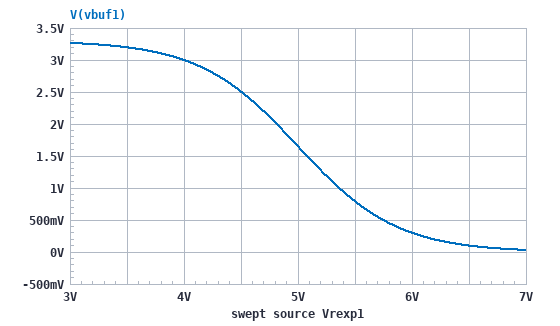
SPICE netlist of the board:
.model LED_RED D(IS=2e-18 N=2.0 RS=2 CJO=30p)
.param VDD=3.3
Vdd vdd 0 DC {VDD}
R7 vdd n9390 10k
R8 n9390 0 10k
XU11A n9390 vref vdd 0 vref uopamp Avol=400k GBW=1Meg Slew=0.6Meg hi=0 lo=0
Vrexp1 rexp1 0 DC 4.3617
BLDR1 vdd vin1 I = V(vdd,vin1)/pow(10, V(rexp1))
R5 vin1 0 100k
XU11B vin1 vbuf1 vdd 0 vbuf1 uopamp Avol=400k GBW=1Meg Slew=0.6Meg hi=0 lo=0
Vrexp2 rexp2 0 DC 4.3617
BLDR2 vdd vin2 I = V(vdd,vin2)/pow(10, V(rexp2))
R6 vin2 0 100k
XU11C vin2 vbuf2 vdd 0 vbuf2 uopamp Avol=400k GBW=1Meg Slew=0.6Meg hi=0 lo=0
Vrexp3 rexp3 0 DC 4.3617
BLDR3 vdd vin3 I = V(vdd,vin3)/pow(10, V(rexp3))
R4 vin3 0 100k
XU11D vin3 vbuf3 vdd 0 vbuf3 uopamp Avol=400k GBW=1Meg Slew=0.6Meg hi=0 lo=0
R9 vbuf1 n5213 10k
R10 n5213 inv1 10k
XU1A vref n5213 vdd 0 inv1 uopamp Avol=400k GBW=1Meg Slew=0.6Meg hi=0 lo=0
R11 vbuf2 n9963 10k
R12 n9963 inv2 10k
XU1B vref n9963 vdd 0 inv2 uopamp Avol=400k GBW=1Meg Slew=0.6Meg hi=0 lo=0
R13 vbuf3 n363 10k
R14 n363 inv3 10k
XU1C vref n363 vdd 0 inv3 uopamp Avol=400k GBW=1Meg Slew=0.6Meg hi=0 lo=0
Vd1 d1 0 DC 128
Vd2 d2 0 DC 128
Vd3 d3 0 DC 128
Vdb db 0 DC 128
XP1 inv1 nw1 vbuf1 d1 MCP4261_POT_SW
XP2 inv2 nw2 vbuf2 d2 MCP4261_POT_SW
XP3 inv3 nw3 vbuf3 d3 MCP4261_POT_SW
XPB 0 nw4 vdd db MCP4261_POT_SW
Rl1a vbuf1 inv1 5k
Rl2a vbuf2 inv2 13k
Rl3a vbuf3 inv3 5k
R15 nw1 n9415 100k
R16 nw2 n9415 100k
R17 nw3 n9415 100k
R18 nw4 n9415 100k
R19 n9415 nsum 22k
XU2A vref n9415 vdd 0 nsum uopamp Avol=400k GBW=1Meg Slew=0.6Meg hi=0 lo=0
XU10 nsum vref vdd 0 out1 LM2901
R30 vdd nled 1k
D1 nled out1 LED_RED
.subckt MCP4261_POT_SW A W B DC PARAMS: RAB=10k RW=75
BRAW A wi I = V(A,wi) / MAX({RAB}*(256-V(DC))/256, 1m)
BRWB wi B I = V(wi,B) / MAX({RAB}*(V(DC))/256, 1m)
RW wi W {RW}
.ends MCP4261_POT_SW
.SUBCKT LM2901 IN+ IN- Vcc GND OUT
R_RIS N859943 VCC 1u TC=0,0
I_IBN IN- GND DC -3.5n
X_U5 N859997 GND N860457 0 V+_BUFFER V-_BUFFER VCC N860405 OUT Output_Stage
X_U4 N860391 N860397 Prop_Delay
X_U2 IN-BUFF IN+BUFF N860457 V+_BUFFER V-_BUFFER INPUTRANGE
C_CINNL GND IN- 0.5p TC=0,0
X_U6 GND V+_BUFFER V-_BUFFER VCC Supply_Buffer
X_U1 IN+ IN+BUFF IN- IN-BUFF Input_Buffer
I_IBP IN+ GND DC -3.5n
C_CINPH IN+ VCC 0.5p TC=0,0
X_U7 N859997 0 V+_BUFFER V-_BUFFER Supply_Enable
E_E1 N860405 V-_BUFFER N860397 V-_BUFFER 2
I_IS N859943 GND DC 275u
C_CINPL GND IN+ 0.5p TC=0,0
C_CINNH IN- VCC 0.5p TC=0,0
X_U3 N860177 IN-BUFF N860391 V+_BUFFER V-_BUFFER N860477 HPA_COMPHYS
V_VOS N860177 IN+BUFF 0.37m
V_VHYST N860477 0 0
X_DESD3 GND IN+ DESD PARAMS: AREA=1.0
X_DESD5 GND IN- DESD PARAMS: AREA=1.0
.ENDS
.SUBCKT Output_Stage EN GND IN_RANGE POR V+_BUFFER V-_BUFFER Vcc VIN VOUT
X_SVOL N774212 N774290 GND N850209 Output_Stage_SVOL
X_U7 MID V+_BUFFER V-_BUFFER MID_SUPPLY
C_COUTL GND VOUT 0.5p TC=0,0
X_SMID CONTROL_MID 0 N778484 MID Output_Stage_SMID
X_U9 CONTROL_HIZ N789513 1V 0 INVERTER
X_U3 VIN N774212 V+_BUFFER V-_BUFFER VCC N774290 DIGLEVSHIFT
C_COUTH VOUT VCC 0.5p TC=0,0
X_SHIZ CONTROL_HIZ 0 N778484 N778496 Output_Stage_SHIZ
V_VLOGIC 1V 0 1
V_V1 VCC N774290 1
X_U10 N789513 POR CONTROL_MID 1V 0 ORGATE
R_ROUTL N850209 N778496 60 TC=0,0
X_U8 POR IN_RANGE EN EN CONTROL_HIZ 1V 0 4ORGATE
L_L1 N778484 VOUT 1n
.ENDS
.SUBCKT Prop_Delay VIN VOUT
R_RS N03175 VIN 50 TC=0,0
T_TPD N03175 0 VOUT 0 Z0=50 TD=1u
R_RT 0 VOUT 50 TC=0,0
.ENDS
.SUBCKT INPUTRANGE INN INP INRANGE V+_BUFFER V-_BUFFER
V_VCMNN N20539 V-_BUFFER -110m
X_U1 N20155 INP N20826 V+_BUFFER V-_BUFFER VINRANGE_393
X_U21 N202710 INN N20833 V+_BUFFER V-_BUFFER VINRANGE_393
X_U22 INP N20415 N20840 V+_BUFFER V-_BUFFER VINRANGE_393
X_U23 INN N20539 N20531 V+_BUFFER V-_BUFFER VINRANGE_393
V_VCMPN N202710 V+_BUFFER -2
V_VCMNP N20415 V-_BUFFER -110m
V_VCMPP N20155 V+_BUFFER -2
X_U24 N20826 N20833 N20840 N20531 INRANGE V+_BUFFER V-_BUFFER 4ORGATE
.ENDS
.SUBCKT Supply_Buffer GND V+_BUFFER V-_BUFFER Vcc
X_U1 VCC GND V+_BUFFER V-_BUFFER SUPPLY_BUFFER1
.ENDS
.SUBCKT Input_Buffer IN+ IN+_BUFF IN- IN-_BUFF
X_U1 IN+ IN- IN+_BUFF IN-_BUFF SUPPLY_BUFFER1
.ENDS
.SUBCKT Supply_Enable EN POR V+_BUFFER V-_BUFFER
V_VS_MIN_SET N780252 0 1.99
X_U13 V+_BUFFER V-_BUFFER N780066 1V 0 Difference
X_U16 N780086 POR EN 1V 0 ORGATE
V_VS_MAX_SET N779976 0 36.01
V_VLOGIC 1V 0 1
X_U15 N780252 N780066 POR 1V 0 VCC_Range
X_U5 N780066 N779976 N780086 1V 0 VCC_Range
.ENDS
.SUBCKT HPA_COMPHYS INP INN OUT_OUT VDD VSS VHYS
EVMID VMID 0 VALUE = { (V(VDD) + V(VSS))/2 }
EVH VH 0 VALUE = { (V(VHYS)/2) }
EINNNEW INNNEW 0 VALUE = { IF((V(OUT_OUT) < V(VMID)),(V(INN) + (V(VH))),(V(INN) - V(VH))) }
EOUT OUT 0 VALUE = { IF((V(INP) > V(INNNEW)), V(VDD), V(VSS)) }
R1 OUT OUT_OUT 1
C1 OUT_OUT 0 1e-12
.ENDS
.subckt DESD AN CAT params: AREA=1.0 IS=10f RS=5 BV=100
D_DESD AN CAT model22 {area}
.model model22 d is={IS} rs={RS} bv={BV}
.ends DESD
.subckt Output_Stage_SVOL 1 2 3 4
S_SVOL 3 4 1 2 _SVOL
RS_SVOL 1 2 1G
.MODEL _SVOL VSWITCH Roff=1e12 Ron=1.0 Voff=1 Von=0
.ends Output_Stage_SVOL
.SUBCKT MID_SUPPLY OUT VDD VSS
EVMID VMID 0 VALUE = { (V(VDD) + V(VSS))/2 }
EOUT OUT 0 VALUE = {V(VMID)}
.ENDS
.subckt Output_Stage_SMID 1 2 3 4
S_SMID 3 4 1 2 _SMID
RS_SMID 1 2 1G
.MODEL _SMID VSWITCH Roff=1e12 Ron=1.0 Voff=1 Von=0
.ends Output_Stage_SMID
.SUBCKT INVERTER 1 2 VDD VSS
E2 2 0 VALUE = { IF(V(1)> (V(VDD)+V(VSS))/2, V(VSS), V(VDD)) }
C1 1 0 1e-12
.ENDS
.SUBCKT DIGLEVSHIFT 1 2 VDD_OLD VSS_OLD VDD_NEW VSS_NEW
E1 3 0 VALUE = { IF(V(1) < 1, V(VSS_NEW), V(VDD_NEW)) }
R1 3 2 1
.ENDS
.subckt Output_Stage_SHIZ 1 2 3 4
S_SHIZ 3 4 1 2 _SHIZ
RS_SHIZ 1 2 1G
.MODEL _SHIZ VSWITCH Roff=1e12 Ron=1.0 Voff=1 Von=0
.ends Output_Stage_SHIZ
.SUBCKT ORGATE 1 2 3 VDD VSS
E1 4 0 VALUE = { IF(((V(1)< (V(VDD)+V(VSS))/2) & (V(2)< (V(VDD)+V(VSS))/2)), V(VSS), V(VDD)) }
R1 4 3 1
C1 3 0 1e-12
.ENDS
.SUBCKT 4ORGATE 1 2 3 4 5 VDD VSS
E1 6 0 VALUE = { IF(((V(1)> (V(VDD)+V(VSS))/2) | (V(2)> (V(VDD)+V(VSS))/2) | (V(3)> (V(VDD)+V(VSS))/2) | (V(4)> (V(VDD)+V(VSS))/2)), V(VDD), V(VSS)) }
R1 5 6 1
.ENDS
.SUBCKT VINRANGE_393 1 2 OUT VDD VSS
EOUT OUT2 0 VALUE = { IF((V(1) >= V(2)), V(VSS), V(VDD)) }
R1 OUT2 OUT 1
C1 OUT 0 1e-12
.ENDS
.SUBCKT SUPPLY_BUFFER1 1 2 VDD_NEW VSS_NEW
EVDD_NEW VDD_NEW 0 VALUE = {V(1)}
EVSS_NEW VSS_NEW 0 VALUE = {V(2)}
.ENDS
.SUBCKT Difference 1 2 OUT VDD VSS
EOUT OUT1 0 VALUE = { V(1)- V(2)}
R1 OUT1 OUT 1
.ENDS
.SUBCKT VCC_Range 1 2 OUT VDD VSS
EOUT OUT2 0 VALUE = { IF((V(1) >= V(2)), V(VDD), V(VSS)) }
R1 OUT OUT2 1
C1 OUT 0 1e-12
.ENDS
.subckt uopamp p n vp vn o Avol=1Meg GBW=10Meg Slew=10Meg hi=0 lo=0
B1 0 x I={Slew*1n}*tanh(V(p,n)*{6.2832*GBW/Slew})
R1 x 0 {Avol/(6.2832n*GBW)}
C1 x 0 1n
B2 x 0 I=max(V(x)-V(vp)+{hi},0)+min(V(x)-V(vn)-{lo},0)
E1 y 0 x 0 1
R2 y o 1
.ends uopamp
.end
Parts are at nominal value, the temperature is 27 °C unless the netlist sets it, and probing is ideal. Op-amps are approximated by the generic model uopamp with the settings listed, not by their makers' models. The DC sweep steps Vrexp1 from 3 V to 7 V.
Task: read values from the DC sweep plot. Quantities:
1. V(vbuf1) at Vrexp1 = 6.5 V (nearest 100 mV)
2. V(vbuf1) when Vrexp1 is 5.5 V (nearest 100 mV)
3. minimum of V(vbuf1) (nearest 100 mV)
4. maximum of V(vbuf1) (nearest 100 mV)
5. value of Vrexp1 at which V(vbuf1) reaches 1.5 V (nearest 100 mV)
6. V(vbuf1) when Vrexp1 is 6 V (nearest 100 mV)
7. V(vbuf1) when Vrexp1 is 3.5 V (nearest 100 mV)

100 mV
800 mV
0 V
3.3 V
5.1 V
300 mV
3.2 V
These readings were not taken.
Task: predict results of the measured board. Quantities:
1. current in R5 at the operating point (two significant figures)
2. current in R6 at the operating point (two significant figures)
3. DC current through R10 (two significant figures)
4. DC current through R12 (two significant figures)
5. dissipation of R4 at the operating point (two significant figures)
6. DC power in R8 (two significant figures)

27 µA
27 µA
100 µA
100 µA
72 µW
270 µW
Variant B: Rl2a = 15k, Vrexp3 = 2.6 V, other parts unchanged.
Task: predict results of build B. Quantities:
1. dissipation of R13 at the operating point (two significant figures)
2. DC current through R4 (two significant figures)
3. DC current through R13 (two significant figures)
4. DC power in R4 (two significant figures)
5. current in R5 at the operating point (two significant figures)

270 µW
33 µA
160 µA
110 µW
27 µA
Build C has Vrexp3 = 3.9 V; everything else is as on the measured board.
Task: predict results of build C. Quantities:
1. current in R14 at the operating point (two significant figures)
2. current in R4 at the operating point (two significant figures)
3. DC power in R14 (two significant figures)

140 µA
31 µA
200 µW
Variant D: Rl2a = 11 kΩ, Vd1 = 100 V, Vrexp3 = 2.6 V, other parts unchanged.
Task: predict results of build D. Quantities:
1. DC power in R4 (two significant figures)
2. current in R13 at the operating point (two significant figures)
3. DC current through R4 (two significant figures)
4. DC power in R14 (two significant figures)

110 µW
160 µA
33 µA
270 µW
